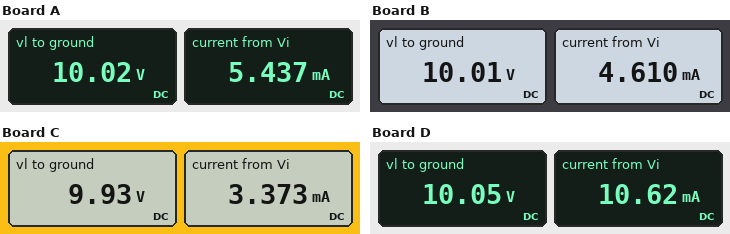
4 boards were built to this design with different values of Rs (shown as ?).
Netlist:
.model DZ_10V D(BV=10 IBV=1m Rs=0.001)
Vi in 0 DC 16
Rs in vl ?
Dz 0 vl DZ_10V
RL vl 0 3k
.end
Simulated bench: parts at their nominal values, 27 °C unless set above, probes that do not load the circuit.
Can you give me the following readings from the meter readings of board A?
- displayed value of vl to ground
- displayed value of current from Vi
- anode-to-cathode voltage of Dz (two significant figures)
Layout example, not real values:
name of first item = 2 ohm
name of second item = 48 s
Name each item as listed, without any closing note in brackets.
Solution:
displayed value of vl to ground = 10.02 V
displayed value of current from Vi = 5.437 mA
anode-to-cathode voltage of Dz = -10 V
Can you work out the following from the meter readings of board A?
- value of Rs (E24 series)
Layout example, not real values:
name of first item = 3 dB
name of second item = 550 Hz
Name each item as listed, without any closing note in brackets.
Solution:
value of Rs = 1.1 kΩ
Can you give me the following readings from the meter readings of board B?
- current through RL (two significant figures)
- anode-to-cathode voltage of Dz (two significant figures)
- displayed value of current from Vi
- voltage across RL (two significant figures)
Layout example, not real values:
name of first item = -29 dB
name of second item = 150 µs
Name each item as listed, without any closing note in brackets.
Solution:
current through RL = 3.3 mA
anode-to-cathode voltage of Dz = -10 V
displayed value of current from Vi = 4.610 mA
voltage across RL = 10 V
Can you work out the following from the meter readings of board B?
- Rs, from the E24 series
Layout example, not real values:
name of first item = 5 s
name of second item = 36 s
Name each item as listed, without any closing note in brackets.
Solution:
Rs, from the E24 series = 1.3 kΩ
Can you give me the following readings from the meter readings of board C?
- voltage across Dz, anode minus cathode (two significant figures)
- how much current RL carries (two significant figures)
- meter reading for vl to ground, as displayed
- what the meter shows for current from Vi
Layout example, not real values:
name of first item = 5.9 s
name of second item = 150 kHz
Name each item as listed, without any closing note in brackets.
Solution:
voltage across Dz, anode minus cathode = -9.9 V
how much current RL carries = 3.3 mA
meter reading for vl to ground, as displayed = 9.93 V
what the meter shows for current from Vi = 3.373 mA
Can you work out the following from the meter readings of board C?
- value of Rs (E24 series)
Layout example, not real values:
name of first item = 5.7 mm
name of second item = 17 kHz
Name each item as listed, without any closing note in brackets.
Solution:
value of Rs = 1.8 kΩ
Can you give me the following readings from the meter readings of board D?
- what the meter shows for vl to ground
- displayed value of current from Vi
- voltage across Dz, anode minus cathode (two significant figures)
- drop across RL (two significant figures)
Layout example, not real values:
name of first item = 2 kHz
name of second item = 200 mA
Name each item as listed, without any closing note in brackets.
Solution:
what the meter shows for vl to ground = 10.05 V
displayed value of current from Vi = 10.62 mA
voltage across Dz, anode minus cathode = -10 V
drop across RL = 10 V
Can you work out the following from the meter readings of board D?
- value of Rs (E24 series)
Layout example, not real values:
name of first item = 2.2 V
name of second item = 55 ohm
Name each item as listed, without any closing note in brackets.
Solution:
value of Rs = 560 Ω
